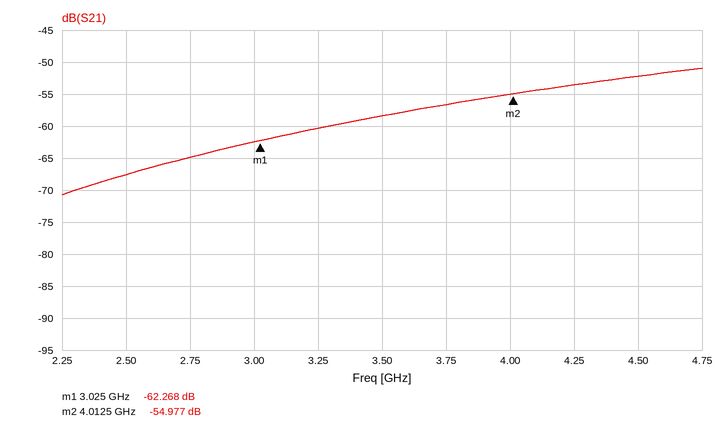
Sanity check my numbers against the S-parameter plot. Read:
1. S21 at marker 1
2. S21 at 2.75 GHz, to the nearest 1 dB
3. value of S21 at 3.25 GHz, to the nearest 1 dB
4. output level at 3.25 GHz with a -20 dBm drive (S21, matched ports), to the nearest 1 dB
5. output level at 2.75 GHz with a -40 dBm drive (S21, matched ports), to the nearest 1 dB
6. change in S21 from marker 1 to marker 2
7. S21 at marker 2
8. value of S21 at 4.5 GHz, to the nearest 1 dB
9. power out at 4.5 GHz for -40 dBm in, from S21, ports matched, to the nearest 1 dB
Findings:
-62.268 dB
-65 dB
-60 dB
-80 dBm
-105 dBm
7.291 dB
-54.977 dB
-52 dB
-92 dBm
